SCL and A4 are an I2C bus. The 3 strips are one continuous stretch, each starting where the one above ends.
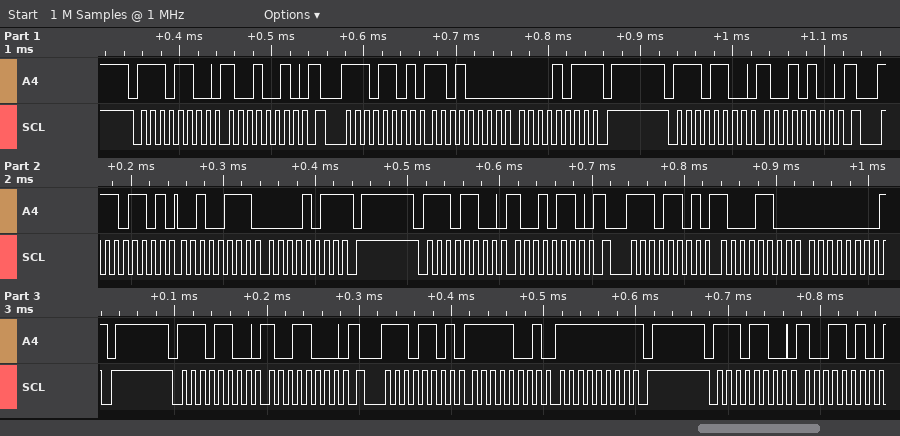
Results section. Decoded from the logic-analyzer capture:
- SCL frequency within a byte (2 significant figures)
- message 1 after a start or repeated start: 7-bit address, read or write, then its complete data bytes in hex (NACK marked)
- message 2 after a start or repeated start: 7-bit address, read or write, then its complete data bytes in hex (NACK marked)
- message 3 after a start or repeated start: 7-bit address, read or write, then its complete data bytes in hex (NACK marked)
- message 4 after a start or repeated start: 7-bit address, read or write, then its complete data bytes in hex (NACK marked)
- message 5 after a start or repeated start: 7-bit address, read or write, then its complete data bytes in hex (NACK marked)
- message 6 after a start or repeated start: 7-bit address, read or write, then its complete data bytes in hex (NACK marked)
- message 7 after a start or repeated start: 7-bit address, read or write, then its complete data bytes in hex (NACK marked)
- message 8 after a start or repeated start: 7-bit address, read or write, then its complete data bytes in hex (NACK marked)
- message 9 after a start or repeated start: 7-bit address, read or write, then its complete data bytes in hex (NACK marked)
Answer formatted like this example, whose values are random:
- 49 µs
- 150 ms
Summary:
- 100 kHz
- 0x76 write: 92
- 0x76 read: D0 0B NACK
- 0x76 write: 94
- 0x76 read: 27 0B NACK
- 0x76 write: 96
- 0x76 read: 8C 00 NACK
- 0x76 write: 98
- 0x76 read: F9 FF NACK
- 0x76 write: 9A
